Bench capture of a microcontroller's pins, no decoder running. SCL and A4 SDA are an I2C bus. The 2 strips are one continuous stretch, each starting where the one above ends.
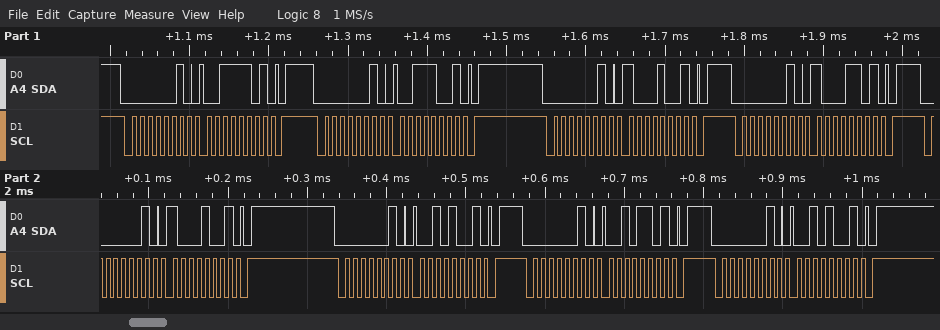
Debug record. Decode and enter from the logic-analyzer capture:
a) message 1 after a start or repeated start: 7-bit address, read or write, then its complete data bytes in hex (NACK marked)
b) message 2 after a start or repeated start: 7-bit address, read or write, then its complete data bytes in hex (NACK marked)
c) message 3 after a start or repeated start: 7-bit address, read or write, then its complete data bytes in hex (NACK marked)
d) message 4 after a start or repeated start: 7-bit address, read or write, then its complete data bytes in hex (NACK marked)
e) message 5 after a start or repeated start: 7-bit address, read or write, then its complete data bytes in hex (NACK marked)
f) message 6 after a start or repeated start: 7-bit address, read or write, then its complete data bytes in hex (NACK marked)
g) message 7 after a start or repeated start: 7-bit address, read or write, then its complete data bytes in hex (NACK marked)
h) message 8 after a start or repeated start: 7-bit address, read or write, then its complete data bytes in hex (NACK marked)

0x01 write: 3D
0x01 write: 39
0x01 write: 89
0x01 write: 8D
0x01 write: 89
0x01 write: 29
0x01 write: 2D
0x01 write: 29
